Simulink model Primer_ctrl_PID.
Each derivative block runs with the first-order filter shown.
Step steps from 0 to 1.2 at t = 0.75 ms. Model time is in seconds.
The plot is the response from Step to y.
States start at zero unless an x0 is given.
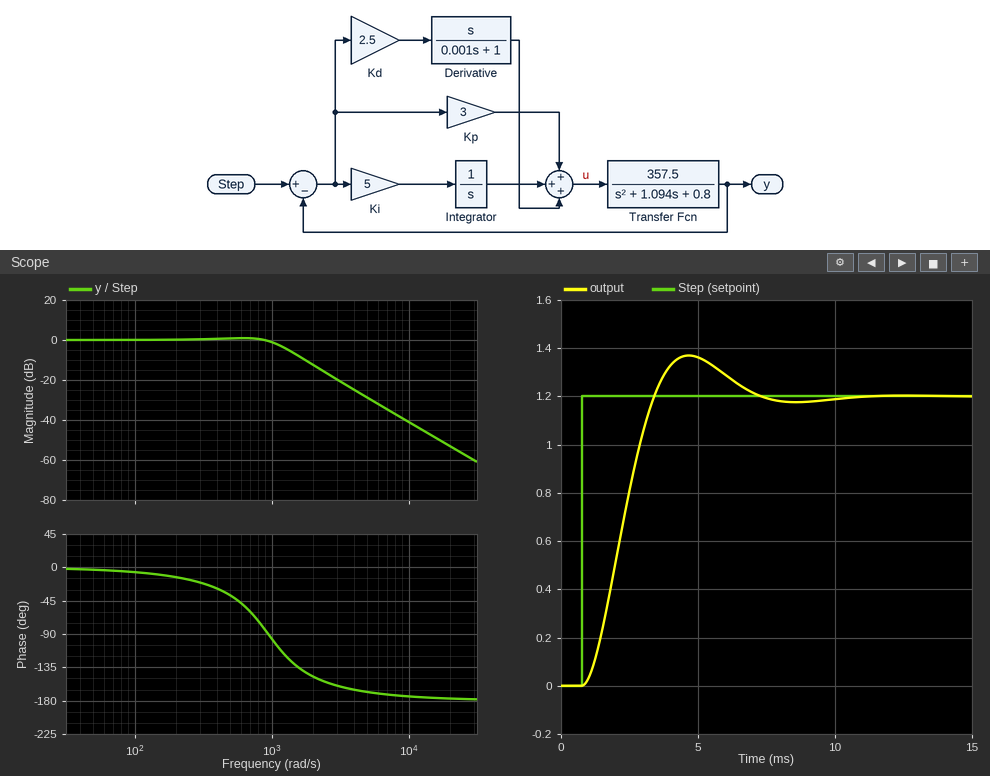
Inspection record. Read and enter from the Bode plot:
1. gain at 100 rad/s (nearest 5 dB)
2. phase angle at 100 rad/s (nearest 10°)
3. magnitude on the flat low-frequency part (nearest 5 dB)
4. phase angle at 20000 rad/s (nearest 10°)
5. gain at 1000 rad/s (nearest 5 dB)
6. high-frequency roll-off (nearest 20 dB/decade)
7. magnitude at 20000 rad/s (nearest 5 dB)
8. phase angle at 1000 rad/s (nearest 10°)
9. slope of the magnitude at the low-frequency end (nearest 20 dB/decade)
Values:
0 dB
-10°
0 dB
-180°
0 dB
-40 dB/decade
-55 dB
-100°
0 dB/decade
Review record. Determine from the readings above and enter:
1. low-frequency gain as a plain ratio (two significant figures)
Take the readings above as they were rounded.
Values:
1.0
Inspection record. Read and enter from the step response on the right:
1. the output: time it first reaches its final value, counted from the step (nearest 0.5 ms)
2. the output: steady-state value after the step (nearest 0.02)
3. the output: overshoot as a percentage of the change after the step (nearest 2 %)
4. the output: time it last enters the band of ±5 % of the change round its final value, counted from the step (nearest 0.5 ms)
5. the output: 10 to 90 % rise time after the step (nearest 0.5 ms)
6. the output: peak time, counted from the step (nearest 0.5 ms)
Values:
2.5 ms
1.20
14 %
5.5 ms
2.0 ms
4.0 ms
